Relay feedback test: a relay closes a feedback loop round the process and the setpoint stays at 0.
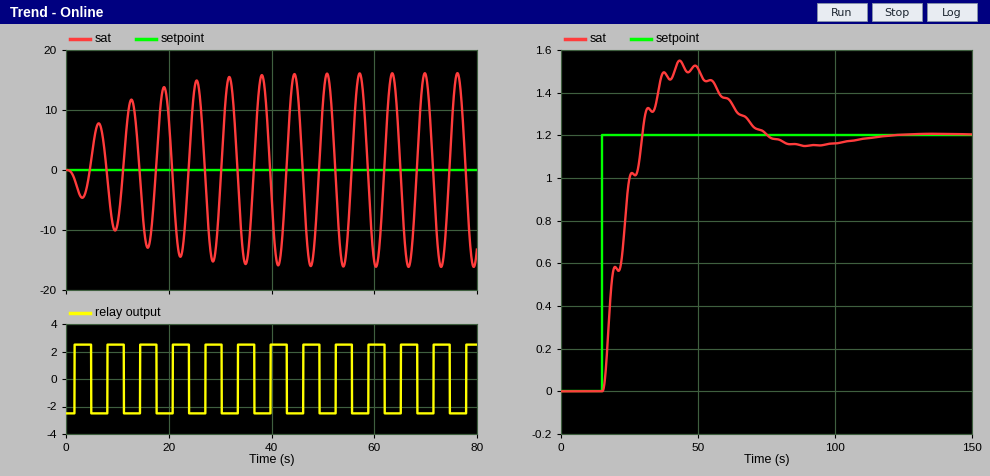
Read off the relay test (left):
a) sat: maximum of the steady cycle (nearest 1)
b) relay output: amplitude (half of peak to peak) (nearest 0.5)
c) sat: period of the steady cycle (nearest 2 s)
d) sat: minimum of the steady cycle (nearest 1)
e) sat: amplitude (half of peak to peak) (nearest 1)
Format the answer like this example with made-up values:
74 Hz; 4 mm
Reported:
16; 2.5; 6 s; -16; 16
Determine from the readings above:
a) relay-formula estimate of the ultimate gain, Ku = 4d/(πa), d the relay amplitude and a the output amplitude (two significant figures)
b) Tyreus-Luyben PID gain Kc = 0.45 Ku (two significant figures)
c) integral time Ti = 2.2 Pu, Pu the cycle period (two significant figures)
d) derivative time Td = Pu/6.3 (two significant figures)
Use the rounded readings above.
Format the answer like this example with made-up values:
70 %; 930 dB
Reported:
0.20; 0.090; 13 s; 0.95 s
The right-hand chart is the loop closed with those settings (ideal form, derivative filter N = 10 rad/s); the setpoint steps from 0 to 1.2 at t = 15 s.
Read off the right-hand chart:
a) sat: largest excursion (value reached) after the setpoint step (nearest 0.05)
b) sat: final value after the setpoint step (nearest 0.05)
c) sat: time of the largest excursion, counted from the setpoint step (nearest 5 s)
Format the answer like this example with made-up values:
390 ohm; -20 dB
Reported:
1.55; 1.20; 30 s
